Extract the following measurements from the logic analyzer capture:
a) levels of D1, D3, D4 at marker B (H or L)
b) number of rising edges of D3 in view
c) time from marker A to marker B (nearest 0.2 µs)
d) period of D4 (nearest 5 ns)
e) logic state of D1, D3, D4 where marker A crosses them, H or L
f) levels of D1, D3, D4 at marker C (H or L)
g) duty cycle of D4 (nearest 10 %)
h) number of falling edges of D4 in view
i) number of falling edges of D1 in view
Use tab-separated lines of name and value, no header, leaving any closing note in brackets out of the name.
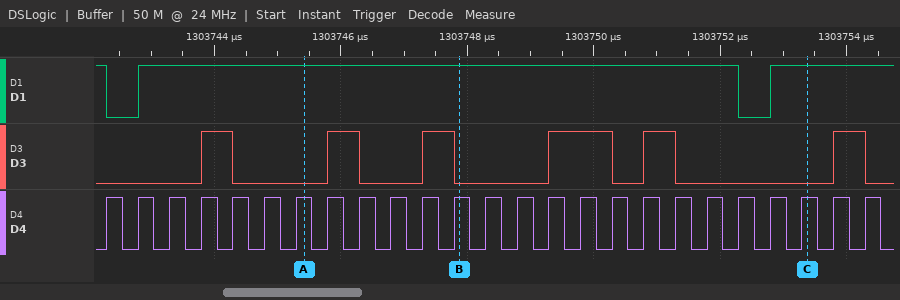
levels of D1, D3, D4 at marker B	D1=H, D3=L, D4=H
number of rising edges of D3 in view	6
time from marker A to marker B	2.4 µs
period of D4	500 ns
logic state of D1, D3, D4 where marker A crosses them, H or L	D1=H, D3=L, D4=H
levels of D1, D3, D4 at marker C	D1=H, D3=L, D4=H
duty cycle of D4	50 %
number of falling edges of D4 in view	25
number of falling edges of D1 in view	2
